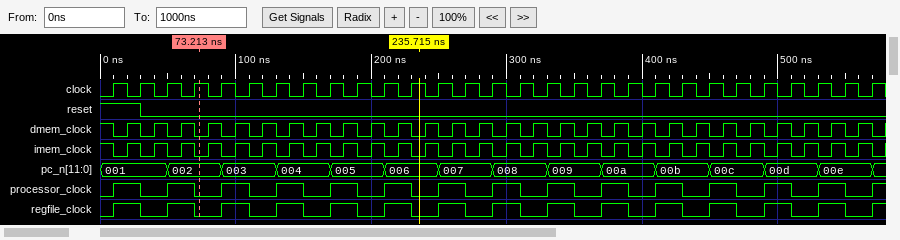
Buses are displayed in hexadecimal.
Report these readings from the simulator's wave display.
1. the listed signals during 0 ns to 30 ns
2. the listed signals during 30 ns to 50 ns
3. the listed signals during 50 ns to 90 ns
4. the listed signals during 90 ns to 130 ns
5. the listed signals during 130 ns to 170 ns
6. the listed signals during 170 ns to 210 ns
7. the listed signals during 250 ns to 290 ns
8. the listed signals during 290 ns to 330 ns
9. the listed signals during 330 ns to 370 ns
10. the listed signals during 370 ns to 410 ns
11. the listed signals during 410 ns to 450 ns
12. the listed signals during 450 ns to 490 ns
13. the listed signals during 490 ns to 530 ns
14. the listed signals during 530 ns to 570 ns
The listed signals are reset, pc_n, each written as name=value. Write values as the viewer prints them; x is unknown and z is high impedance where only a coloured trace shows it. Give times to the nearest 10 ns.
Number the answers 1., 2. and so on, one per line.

1. reset=1, pc_n=001
2. reset=0, pc_n=001
3. reset=0, pc_n=002
4. reset=0, pc_n=003
5. reset=0, pc_n=004
6. reset=0, pc_n=005
7. reset=0, pc_n=007
8. reset=0, pc_n=008
9. reset=0, pc_n=009
10. reset=0, pc_n=00a
11. reset=0, pc_n=00b
12. reset=0, pc_n=00c
13. reset=0, pc_n=00d
14. reset=0, pc_n=00e
